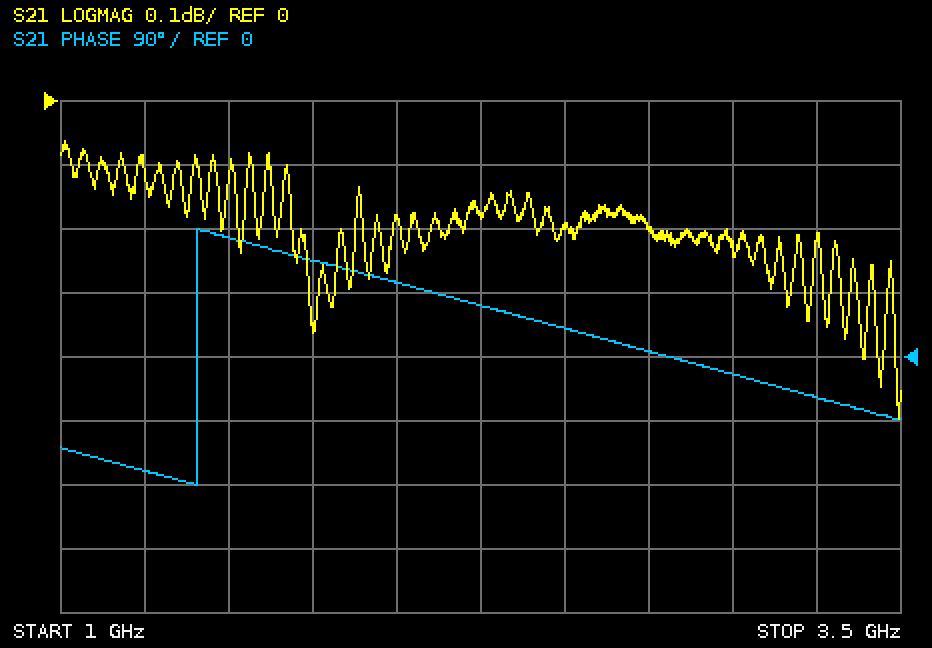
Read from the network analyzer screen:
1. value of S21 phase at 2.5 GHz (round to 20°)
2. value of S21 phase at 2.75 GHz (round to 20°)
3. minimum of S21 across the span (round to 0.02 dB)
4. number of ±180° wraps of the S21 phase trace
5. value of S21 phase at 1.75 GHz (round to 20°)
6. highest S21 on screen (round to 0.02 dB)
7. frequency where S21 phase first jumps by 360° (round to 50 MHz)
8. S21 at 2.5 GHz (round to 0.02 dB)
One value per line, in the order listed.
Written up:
40°
0°
-0.50 dB
1
140°
-0.06 dB
1.40 GHz
-0.20 dB
